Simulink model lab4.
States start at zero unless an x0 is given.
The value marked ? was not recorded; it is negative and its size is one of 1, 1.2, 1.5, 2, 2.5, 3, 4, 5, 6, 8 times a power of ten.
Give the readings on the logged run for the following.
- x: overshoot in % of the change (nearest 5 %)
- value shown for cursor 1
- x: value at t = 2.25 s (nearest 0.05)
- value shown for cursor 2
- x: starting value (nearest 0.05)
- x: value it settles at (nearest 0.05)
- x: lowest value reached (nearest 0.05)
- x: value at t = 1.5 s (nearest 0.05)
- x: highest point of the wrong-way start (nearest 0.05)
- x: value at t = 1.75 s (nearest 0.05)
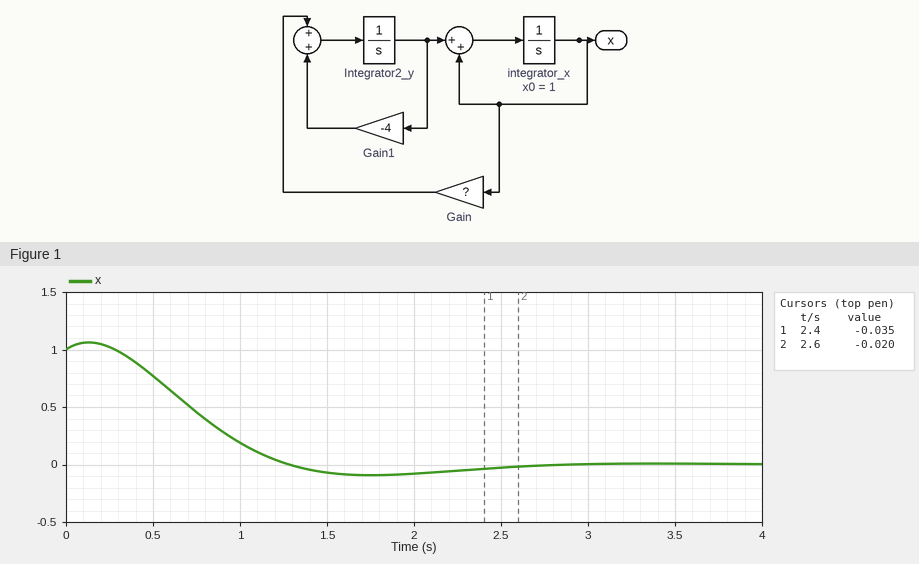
10 %
-0.035
-0.05
-0.020
1.00
0.00
-0.10
-0.05
1.05
-0.10
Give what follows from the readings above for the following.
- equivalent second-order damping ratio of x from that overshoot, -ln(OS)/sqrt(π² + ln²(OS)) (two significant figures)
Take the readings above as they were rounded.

0.59
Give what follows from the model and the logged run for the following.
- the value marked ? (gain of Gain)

-10
